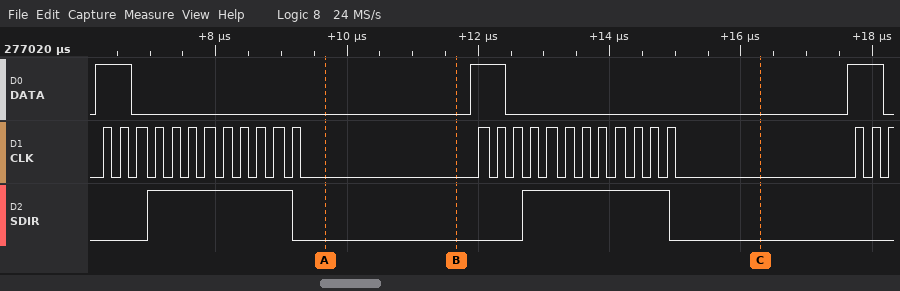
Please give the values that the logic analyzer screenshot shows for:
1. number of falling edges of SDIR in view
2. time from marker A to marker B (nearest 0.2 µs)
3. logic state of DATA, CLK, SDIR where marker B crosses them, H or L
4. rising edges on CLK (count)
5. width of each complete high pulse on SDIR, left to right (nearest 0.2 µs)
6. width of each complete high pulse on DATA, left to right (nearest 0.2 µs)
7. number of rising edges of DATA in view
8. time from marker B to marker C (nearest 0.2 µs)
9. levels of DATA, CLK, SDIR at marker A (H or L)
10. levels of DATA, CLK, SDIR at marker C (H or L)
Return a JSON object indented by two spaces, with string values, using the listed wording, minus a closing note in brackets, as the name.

{
  "number of falling edges of SDIR in view": "2",
  "time from marker A to marker B": "2 µs",
  "logic state of DATA, CLK, SDIR where marker B crosses them, H or L": "DATA=L, CLK=L, SDIR=L",
  "rising edges on CLK": "27",
  "width of each complete high pulse on SDIR, left to right": "2.2 µs, 2.2 µs",
  "width of each complete high pulse on DATA, left to right": "0.6 µs, 0.6 µs, 0.6 µs",
  "number of rising edges of DATA in view": "3",
  "time from marker B to marker C": "4.6 µs",
  "levels of DATA, CLK, SDIR at marker A": "DATA=L, CLK=L, SDIR=L",
  "levels of DATA, CLK, SDIR at marker C": "DATA=L, CLK=L, SDIR=L"
}
